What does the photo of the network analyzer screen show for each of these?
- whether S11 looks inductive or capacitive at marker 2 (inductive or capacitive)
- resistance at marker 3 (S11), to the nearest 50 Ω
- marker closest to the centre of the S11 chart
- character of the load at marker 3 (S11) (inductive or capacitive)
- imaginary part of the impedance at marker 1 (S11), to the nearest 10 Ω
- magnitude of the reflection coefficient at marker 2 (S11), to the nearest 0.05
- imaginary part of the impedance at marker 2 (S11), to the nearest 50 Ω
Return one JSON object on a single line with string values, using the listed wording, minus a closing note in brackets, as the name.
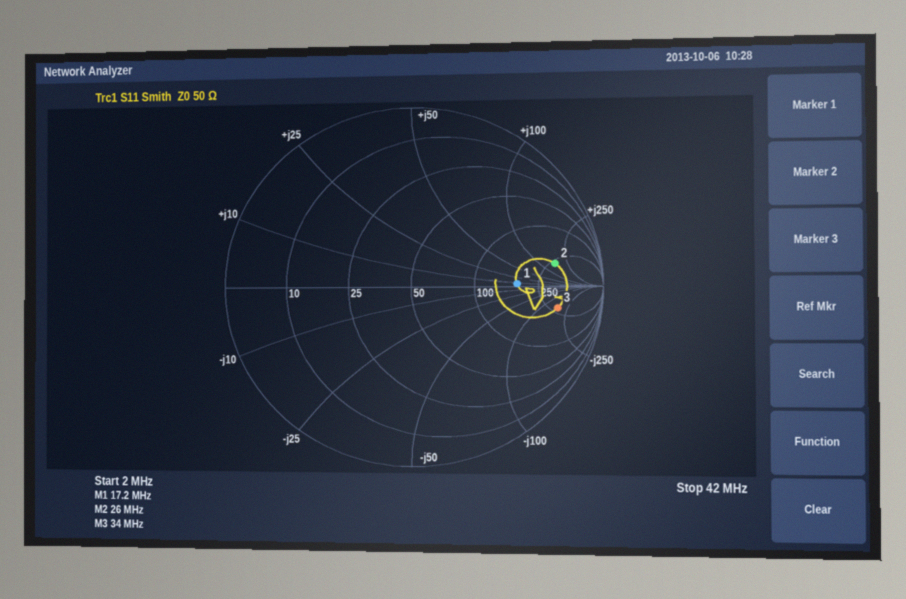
{"whether S11 looks inductive or capacitive at marker 2": "inductive", "resistance at marker 3 (S11), to the nearest 50 Ω": "300 Ω", "marker closest to the centre of the S11 chart": "marker 1", "character of the load at marker 3 (S11)": "capacitive", "imaginary part of the impedance at marker 1 (S11), to the nearest 10 Ω": "+10 Ω", "magnitude of the reflection coefficient at marker 2 (S11), to the nearest 0.05": "0.75", "imaginary part of the impedance at marker 2 (S11), to the nearest 50 Ω": "+150 Ω"}
